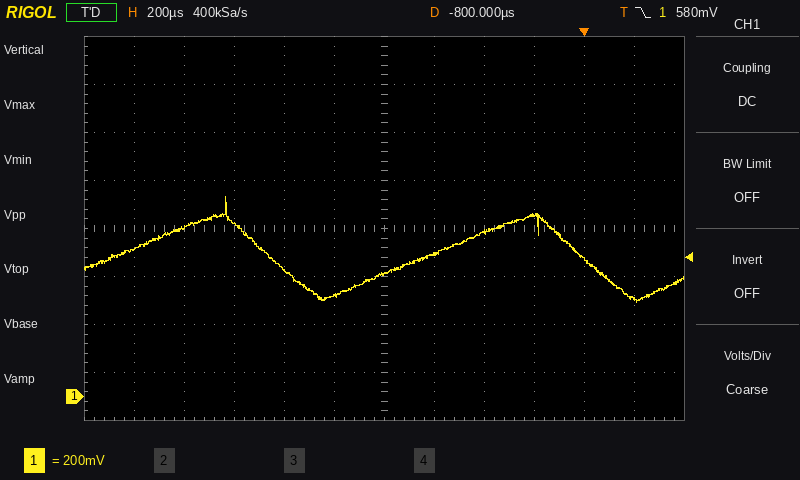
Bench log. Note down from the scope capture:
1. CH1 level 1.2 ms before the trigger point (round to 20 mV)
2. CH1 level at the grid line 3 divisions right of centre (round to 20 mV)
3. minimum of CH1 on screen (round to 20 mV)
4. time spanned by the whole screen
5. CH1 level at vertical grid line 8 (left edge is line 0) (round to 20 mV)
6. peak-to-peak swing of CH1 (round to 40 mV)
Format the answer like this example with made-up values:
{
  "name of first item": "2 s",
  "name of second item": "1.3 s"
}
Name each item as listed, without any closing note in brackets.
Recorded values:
{
  "CH1 level 1.2 ms before the trigger point": "520 mV",
  "CH1 level at the grid line 3 divisions right of centre": "760 mV",
  "minimum of CH1 on screen": "400 mV",
  "time spanned by the whole screen": "2.4 ms",
  "CH1 level at vertical grid line 8 (left edge is line 0)": "680 mV",
  "peak-to-peak swing of CH1": "440 mV"
}
